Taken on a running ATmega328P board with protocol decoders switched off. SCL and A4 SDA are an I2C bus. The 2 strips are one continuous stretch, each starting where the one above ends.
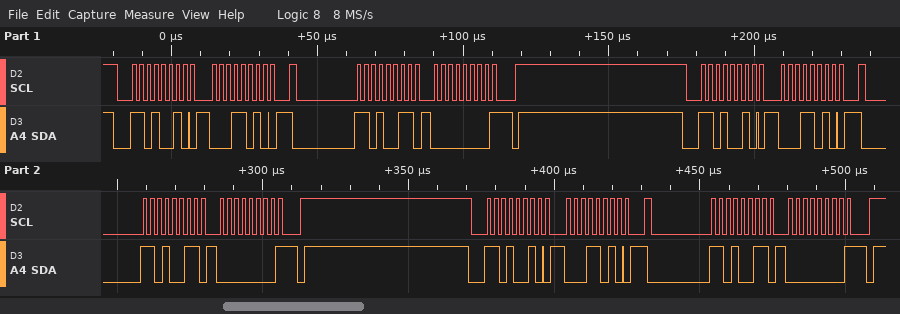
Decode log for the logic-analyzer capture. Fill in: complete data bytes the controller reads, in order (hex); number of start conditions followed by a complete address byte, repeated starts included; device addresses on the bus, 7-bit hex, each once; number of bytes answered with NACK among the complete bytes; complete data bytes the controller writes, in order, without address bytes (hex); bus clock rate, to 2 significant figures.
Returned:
00 00 00
6
0x69
3
1A 1A 1A
400 kHz
